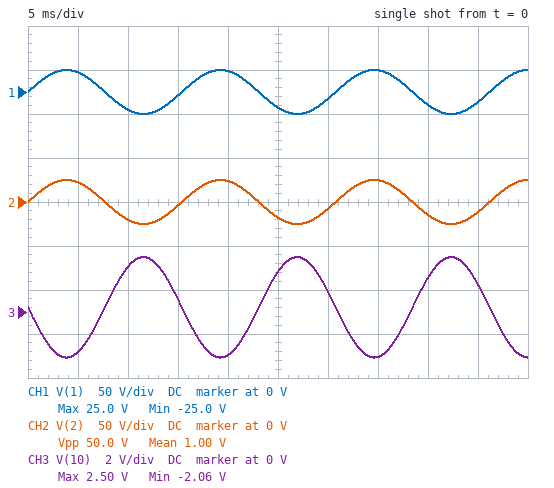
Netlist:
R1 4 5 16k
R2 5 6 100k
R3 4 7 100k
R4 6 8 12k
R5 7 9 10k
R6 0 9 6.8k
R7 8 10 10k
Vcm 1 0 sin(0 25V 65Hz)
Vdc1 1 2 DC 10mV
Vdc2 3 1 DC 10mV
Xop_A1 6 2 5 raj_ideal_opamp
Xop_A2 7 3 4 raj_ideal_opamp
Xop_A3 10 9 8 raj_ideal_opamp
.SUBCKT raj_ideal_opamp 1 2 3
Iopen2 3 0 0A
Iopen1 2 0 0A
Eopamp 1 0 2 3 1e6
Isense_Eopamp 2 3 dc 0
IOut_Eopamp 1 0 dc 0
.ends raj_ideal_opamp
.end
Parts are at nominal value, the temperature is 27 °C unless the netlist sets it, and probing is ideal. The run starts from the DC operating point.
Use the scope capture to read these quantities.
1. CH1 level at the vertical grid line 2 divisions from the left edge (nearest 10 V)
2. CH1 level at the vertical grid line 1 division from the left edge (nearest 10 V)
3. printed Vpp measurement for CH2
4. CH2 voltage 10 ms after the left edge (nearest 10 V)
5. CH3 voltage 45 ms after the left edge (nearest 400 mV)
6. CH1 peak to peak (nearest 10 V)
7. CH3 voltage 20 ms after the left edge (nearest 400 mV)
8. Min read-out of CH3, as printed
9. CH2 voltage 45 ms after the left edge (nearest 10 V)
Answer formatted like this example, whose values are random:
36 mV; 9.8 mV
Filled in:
-20 V; 20 V; 50.0 V; -20 V; 1.2 V; 50 V; -2.0 V; -2.06 V; -10 V
